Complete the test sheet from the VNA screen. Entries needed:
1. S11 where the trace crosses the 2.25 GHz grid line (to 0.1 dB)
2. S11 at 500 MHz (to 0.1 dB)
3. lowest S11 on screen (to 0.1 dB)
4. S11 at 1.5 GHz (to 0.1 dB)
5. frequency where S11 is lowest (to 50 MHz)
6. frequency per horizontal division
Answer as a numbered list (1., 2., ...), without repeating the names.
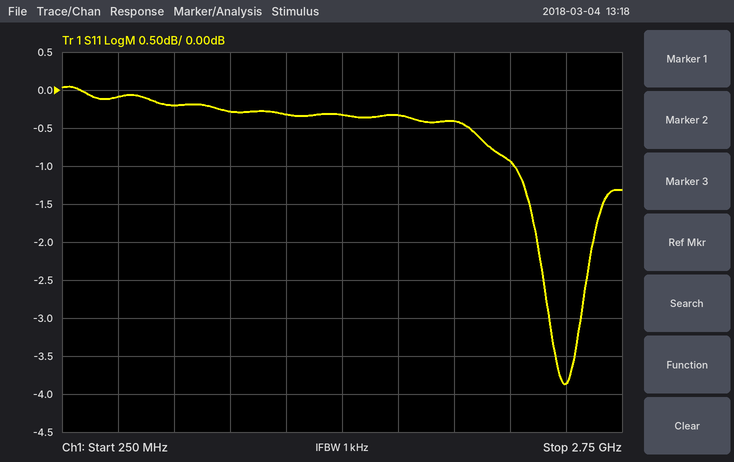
1. -0.9 dB
2. -0.1 dB
3. -3.9 dB
4. -0.3 dB
5. 2.50 GHz
6. 250 MHz
